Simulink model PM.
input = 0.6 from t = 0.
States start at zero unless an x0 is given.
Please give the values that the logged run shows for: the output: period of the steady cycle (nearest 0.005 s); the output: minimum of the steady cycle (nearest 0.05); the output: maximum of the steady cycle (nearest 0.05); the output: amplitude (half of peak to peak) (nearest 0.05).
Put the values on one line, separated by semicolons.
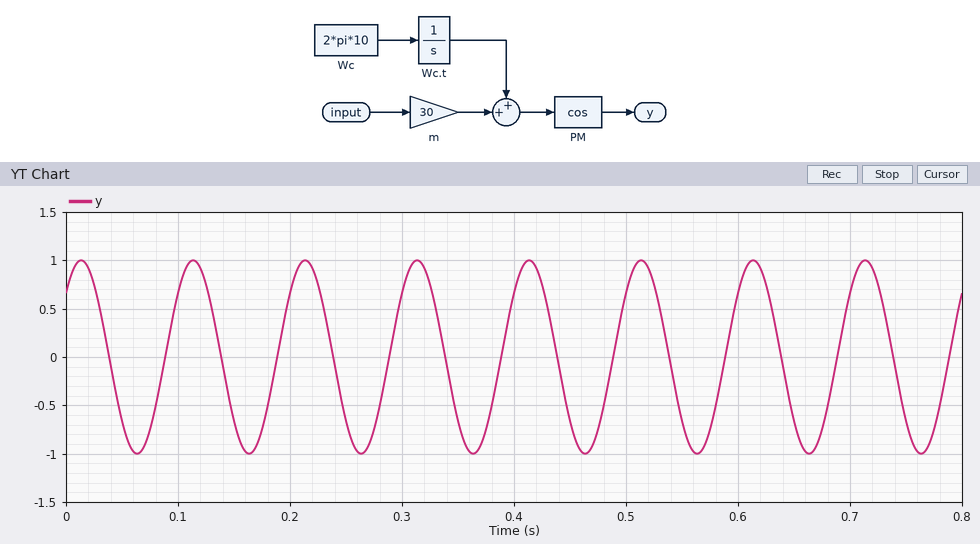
0.100 s; -1.00; 1.00; 1.00
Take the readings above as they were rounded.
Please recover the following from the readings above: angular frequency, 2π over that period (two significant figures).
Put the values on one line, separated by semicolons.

63 rad/s
